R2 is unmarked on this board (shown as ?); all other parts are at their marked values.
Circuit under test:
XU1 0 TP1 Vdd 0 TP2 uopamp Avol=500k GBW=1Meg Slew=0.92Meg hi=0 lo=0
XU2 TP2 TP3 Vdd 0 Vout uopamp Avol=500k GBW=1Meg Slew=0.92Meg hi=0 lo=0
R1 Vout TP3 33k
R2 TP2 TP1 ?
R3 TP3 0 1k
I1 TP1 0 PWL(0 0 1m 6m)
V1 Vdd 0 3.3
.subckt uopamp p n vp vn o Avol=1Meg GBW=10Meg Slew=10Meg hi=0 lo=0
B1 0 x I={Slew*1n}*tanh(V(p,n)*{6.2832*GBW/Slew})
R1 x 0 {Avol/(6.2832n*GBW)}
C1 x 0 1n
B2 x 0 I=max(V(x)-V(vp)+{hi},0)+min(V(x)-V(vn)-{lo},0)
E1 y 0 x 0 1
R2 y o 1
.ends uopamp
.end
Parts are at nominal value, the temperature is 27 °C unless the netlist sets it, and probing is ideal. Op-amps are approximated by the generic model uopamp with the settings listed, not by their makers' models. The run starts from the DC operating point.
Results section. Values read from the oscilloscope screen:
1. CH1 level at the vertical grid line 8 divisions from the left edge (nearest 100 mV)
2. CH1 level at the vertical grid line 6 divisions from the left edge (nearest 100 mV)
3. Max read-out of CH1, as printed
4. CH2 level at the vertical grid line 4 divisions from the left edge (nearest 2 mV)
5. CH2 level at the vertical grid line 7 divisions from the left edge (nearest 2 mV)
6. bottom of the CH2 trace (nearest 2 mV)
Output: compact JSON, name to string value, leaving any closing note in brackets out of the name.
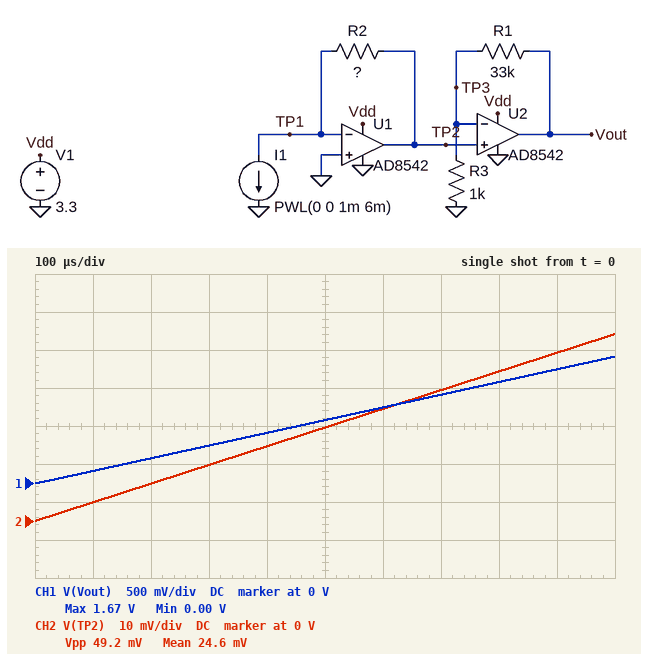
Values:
{"CH1 level at the vertical grid line 8 divisions from the left edge": "1.3 V", "CH1 level at the vertical grid line 6 divisions from the left edge": "1.0 V", "Max read-out of CH1, as printed": "1.67 V", "CH2 level at the vertical grid line 4 divisions from the left edge": "20 mV", "CH2 level at the vertical grid line 7 divisions from the left edge": "34 mV", "bottom of the CH2 trace": "0 V"}
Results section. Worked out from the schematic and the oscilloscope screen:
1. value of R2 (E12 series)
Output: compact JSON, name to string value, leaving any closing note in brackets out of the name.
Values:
{"value of R2": "8.2 Ω"}
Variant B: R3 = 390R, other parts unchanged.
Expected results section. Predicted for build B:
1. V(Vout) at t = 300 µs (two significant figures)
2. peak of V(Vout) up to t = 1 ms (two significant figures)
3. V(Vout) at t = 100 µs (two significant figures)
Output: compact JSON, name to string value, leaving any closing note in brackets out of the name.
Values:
{"V(Vout) at t = 300 µs": "1.2 V", "peak of V(Vout) up to t = 1 ms": "3.3 V", "V(Vout) at t = 100 µs": "360 mV"}
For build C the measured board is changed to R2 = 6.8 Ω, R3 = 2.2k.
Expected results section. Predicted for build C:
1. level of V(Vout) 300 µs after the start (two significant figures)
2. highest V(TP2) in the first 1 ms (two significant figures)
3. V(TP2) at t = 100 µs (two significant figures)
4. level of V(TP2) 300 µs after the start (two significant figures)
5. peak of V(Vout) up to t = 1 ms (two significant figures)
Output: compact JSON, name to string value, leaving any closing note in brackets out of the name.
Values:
{"level of V(Vout) 300 µs after the start": "190 mV", "highest V(TP2) in the first 1 ms": "41 mV", "V(TP2) at t = 100 µs": "4.1 mV", "level of V(TP2) 300 µs after the start": "12 mV", "peak of V(Vout) up to t = 1 ms": "650 mV"}
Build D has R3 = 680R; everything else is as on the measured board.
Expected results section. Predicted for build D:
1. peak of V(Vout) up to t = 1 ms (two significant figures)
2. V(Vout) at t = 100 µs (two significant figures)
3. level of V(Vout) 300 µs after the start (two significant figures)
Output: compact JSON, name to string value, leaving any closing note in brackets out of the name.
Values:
{"peak of V(Vout) up to t = 1 ms": "2.4 V", "V(Vout) at t = 100 µs": "220 mV", "level of V(Vout) 300 µs after the start": "710 mV"}
